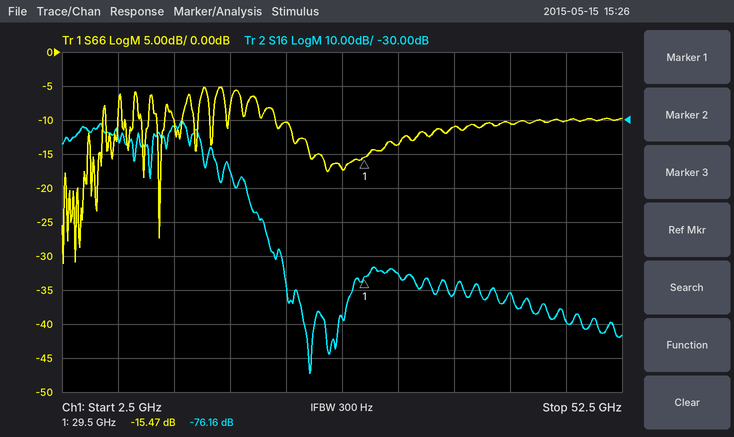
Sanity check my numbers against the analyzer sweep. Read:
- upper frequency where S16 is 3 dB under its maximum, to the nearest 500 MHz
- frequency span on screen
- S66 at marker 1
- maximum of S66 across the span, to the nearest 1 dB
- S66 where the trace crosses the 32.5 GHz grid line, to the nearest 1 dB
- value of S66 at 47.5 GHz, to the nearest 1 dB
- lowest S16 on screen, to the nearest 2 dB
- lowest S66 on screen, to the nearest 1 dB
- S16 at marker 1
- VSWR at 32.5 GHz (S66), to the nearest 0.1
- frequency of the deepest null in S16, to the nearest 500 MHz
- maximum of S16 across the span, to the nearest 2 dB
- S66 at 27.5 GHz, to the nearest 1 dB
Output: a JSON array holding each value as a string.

["13.5 GHz", "50 GHz", "-15.47 dB", "-5 dB", "-14 dB", "-10 dB", "-104 dB", "-31 dB", "-76.16 dB", "1.5", "24.5 GHz", "-30 dB", "-17 dB"]
